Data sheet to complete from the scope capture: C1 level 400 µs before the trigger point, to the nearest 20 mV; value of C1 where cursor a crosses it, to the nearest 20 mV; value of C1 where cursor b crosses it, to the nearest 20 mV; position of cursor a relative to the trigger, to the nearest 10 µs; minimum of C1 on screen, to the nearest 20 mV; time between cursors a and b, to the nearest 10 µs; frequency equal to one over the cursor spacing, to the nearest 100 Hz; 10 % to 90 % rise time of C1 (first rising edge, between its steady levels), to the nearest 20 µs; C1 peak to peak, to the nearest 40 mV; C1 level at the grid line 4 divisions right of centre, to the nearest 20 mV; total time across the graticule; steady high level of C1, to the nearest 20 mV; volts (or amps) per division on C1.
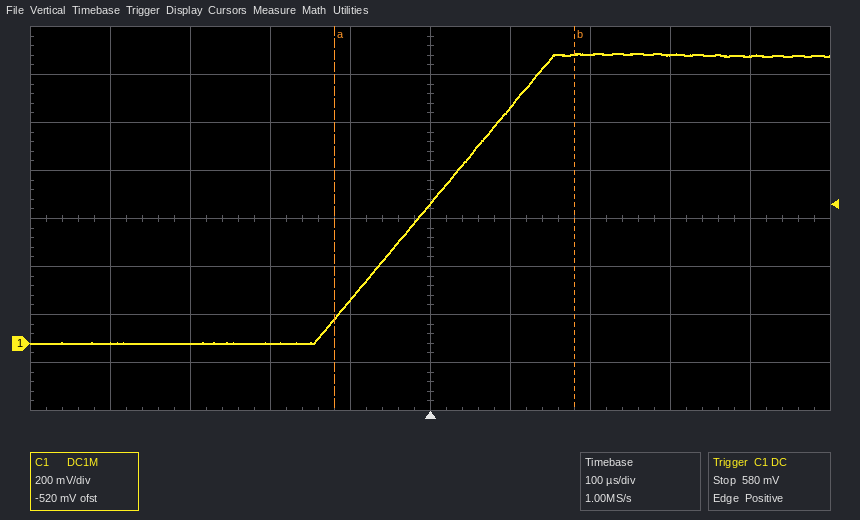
0 mV
100 mV
1.20 V
-120 µs
0 mV
300 µs
3.3 kHz
240 µs
1.20 V
1.20 V
1 ms
1.20 V
200 mV
